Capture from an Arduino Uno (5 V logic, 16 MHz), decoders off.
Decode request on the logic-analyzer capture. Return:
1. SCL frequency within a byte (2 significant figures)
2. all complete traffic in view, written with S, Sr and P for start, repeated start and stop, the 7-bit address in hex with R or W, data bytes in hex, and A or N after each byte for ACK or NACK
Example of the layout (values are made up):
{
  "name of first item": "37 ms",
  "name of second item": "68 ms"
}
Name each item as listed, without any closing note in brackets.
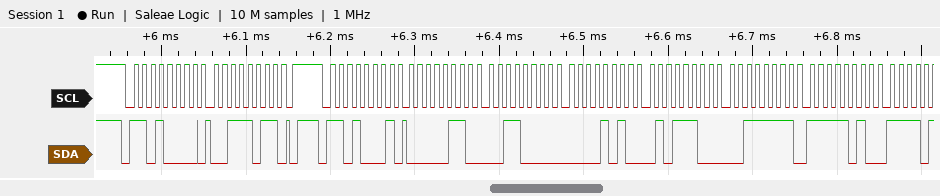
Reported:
{
  "SCL frequency within a byte": "100 kHz",
  "all complete traffic in view, written with S, Sr and P for start, repeated start and stop, the 7-bit address in hex with R or W, data bytes in hex, and A or N after each byte for ACK or NACK": "S 68W A 3B A P S 68R A 06 A 30 A 0A A 5C A 3F A FA A"
}
